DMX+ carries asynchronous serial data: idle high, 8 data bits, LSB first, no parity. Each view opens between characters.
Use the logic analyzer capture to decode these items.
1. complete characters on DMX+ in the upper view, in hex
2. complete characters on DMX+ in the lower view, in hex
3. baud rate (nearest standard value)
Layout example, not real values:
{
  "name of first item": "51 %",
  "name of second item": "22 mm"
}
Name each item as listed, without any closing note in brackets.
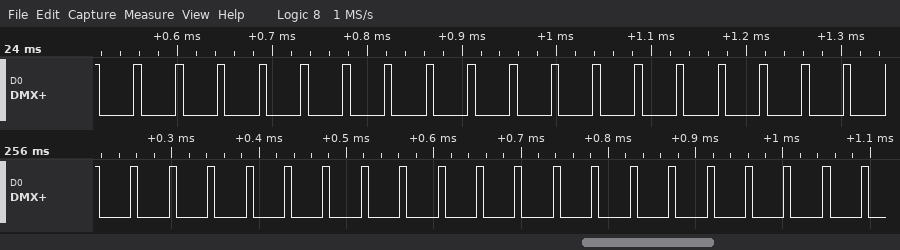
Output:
{
  "complete characters on DMX+ in the upper view, in hex": "08, 08, 08, 08, 08, 08, 08, 08, 08",
  "complete characters on DMX+ in the lower view, in hex": "08, 08, 08, 08, 08, 08, 08, 08, 08, 08",
  "baud rate": "115200 baud"
}
